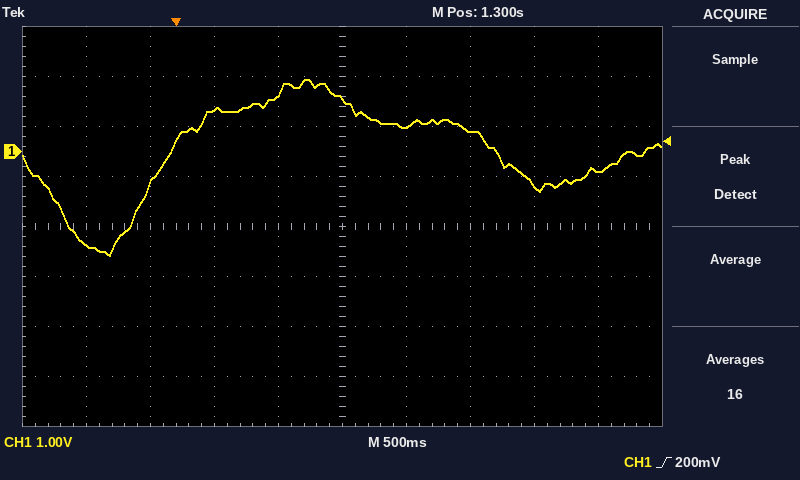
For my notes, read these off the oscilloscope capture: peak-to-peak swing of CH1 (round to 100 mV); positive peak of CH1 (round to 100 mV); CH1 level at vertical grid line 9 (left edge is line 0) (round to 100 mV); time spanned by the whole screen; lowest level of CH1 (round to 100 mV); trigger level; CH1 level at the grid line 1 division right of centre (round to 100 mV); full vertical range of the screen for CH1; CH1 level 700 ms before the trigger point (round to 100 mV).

3.5 V
1.4 V
-400 mV
5 s
-2.1 V
200 mV
500 mV
8 V
-1.9 V
